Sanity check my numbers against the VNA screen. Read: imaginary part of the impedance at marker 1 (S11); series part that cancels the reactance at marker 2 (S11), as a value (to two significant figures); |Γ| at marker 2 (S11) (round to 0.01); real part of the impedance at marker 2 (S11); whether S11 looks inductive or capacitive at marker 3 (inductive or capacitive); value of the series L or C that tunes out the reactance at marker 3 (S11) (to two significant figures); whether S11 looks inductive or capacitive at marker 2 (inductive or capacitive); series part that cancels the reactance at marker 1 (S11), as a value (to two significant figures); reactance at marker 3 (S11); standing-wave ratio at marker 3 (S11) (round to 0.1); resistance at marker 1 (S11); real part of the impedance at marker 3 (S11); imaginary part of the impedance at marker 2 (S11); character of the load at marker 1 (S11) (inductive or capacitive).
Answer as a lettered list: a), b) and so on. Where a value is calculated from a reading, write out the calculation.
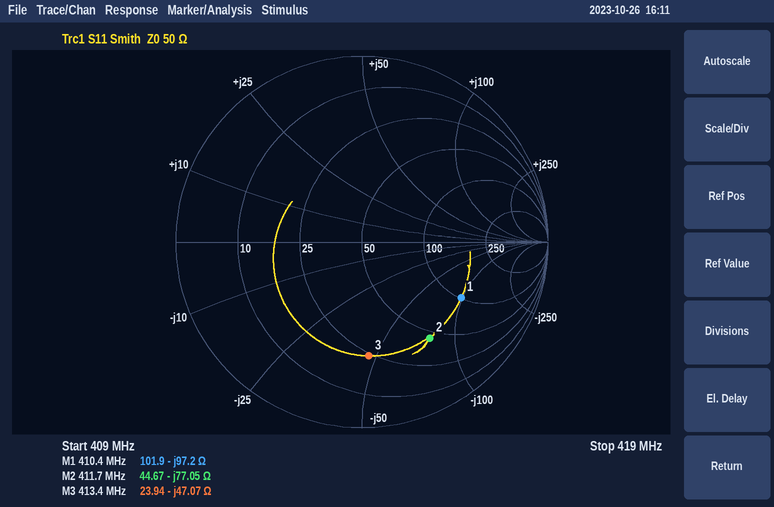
a) -97.2 Ω
b) L = 77.05 Ω/(2π × 411.7 MHz) ≈ 30 nH
c) 0.63
d) 44.67 Ω
e) capacitive
f) L = 47.07 Ω/(2π × 413.4 MHz) ≈ 18 nH
g) capacitive
h) L = 97.2 Ω/(2π × 410.4 MHz) ≈ 38 nH
i) -47.07 Ω
j) 4.2
k) 101.9 Ω
l) 23.94 Ω
m) -77.05 Ω
n) capacitive
